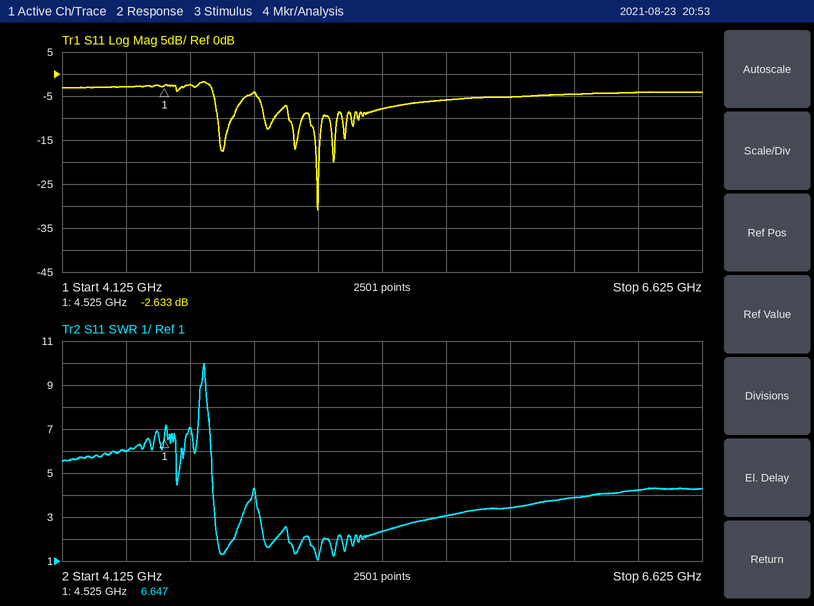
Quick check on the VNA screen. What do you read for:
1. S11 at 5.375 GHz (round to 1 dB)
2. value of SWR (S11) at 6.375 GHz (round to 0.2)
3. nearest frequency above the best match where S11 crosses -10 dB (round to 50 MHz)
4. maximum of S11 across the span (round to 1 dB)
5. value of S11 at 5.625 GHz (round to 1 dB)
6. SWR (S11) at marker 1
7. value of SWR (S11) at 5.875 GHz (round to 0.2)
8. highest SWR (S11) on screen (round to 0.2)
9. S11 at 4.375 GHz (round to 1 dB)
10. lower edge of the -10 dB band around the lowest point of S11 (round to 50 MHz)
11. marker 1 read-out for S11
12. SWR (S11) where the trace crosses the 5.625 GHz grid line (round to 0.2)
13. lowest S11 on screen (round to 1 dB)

-8 dB
4.2
5.15 GHz
-2 dB
-6 dB
6.647
3.4
10.0
-3 dB
5.10 GHz
-2.633 dB
3.0
-31 dB
